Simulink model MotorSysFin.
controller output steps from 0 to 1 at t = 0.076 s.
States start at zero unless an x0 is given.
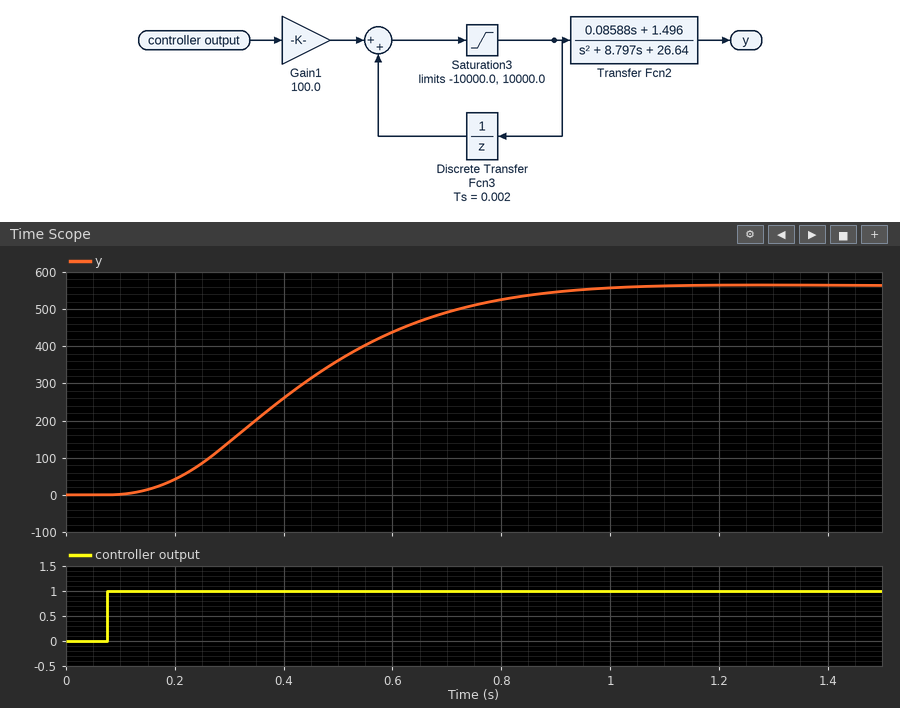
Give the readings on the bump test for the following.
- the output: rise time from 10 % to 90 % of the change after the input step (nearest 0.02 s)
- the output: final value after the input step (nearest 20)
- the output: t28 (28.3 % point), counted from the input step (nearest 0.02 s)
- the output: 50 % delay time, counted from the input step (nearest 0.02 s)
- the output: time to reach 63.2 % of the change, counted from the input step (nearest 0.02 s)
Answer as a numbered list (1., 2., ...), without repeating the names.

1. 0.52 s
2. 560
3. 0.24 s
4. 0.34 s
5. 0.42 s
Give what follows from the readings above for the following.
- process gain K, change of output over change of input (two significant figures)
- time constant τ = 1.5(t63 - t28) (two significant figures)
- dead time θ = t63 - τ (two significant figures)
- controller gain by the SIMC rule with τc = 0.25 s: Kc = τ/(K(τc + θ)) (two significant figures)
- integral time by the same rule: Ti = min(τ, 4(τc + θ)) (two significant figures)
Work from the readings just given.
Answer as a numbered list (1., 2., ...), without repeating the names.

1. 560
2. 0.27 s
3. 0.15 s
4. 0.0012
5. 0.27 s
